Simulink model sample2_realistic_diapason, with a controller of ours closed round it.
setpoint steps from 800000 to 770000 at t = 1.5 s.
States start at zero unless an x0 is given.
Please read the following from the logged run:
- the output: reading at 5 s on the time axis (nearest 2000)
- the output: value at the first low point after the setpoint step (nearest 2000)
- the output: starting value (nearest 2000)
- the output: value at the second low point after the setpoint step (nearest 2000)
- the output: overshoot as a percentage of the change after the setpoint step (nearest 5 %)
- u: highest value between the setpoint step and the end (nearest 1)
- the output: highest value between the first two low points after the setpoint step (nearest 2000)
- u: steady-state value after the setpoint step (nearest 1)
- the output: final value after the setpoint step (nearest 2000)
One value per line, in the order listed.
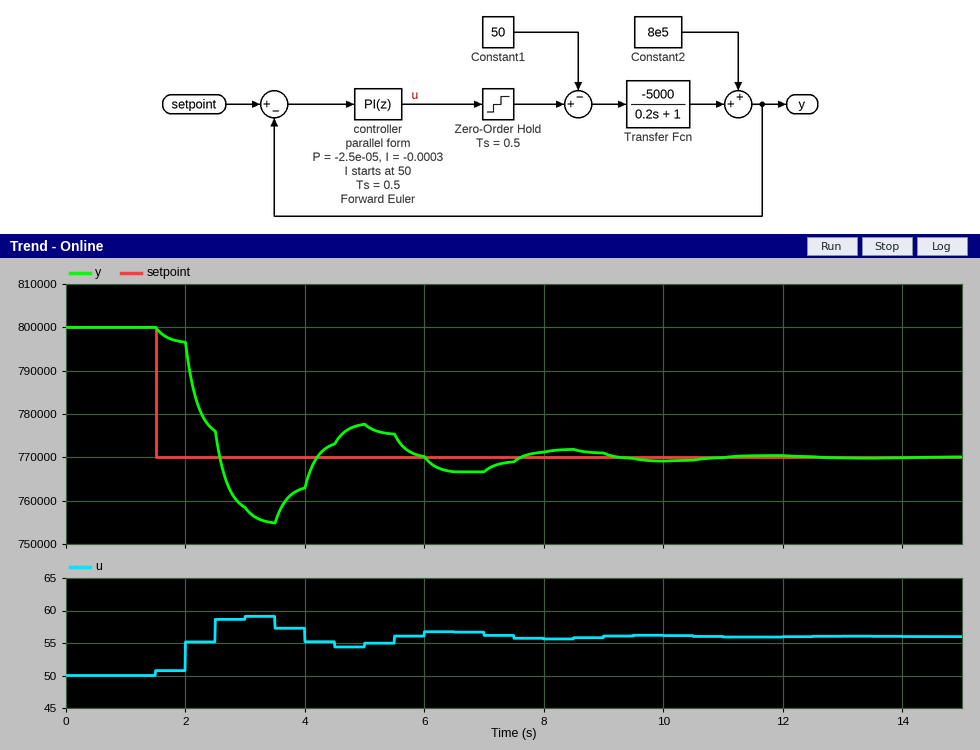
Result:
778000
754000
800000
766000
50 %
59
778000
56
770000
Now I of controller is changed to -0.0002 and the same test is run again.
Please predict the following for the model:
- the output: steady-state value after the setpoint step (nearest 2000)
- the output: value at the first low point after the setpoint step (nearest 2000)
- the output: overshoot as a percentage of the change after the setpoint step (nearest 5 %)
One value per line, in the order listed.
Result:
770000
766000
15 %
